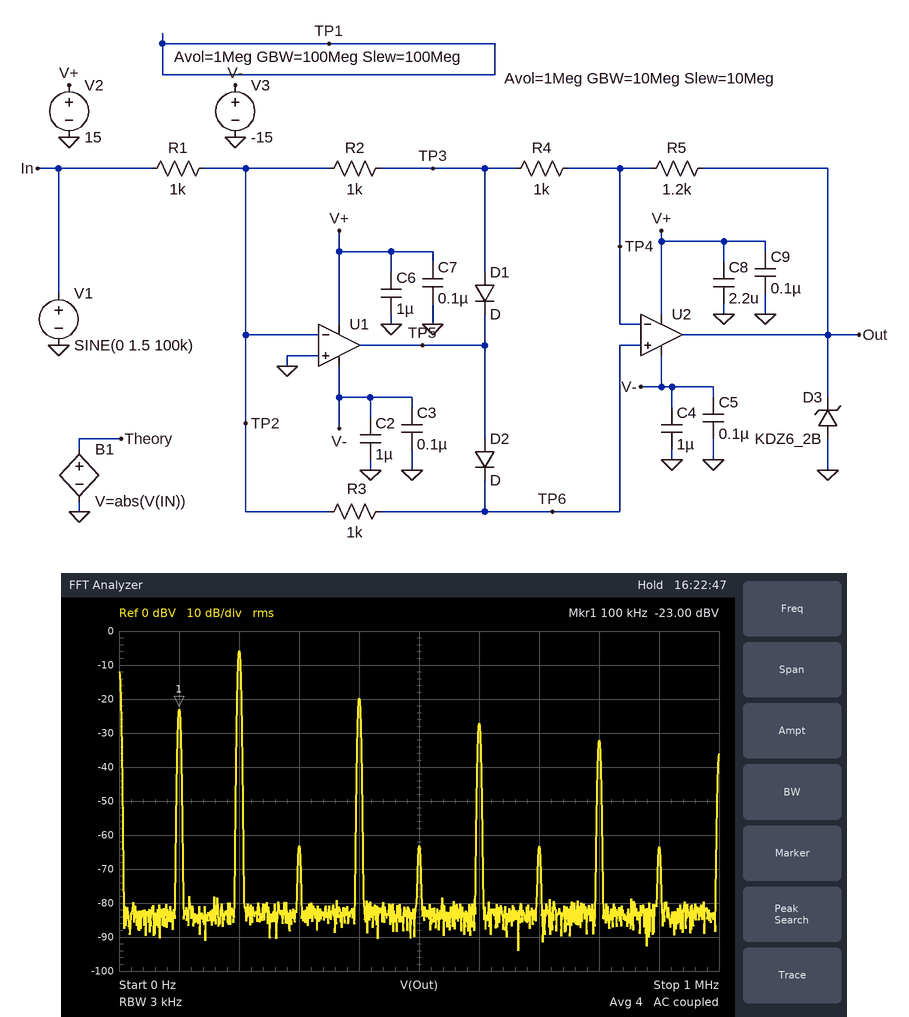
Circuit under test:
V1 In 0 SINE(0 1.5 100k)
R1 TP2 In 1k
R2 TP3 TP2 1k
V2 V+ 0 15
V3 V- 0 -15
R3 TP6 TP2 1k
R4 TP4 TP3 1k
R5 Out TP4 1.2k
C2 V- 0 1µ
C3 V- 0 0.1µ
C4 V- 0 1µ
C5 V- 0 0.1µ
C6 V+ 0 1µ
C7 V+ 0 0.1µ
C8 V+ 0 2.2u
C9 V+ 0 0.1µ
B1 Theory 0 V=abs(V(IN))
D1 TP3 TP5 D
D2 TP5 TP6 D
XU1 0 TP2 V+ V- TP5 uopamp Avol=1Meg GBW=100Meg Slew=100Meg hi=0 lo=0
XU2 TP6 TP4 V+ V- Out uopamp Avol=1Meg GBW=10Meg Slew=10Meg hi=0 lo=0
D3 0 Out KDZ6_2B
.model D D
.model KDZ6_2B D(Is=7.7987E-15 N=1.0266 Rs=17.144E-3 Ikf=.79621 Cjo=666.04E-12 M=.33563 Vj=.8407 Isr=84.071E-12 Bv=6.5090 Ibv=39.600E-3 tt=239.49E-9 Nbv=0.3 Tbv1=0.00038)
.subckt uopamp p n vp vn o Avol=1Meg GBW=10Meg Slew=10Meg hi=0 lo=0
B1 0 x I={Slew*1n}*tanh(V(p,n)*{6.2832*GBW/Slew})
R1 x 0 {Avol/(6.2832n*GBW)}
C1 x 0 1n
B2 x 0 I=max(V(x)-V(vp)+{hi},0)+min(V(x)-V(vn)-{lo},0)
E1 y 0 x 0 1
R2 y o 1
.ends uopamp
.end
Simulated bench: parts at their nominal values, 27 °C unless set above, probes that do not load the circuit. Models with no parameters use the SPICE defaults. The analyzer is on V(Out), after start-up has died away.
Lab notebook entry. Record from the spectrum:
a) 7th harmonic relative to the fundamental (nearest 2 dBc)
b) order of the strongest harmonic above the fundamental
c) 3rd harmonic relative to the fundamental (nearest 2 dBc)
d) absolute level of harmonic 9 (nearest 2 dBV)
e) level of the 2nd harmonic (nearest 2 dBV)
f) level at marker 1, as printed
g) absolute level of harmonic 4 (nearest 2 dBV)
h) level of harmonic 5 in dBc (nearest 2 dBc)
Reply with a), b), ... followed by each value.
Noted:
a) -40 dBc
b) 2
c) -40 dBc
d) -64 dBV
e) -6 dBV
f) -23.00 dBV
g) -20 dBV
h) -40 dBc
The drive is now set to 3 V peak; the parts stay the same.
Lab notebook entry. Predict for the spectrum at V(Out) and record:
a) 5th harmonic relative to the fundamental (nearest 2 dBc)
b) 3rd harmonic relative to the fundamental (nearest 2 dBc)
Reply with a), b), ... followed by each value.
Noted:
a) -44 dBc
b) -44 dBc
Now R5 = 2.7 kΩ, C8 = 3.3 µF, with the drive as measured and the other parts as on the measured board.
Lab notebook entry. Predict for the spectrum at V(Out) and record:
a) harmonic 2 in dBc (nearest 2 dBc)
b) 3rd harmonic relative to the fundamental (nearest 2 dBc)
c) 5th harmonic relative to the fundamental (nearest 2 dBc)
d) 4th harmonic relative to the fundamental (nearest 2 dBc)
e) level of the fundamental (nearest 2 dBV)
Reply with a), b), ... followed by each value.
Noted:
a) 4 dBc
b) -56 dBc
c) -54 dBc
d) -10 dBc
e) -4 dBV
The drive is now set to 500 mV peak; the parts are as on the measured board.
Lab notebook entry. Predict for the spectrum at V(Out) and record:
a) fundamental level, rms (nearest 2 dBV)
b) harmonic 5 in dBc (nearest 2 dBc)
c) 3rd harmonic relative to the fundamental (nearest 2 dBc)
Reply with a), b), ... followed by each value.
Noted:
a) -32 dBV
b) -32 dBc
c) -32 dBc
